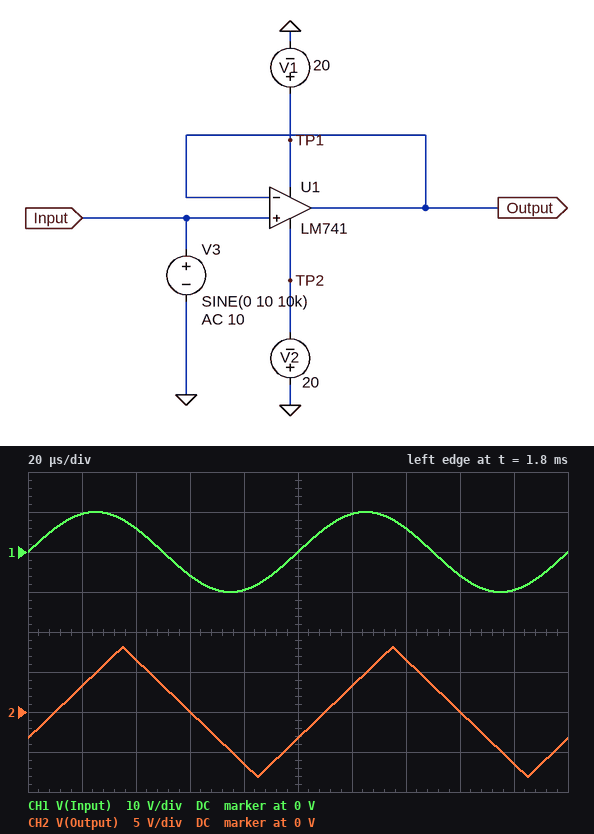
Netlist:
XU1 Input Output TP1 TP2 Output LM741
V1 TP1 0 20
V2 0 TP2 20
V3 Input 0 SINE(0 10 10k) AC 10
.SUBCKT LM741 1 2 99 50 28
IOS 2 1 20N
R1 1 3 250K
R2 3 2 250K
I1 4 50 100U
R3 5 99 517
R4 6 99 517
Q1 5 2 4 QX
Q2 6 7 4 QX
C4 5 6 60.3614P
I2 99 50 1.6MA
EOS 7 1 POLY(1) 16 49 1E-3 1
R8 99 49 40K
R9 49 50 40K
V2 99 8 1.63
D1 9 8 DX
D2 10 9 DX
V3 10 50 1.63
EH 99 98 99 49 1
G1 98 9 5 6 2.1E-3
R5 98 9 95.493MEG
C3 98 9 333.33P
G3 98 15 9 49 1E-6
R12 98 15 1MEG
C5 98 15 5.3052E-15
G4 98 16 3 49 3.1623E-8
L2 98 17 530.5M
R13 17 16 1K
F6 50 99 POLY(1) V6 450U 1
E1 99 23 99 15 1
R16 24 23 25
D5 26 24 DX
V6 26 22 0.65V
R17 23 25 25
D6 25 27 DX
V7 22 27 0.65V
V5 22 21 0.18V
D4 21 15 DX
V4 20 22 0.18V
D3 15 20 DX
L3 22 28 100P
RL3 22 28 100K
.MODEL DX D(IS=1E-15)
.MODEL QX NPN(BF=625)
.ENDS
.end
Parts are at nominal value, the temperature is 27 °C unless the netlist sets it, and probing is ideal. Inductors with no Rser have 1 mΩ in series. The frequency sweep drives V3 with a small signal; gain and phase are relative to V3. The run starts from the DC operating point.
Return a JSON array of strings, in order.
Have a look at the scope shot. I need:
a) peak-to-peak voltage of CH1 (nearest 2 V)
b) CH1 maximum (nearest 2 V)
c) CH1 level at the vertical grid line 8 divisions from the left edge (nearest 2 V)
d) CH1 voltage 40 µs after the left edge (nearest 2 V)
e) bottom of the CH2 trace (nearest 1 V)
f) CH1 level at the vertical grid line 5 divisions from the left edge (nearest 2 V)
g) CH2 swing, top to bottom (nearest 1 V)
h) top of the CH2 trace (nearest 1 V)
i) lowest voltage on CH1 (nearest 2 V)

["20 V", "10 V", "-6 V", "6 V", "-8 V", "0 V", "16 V", "8 V", "-10 V"]
